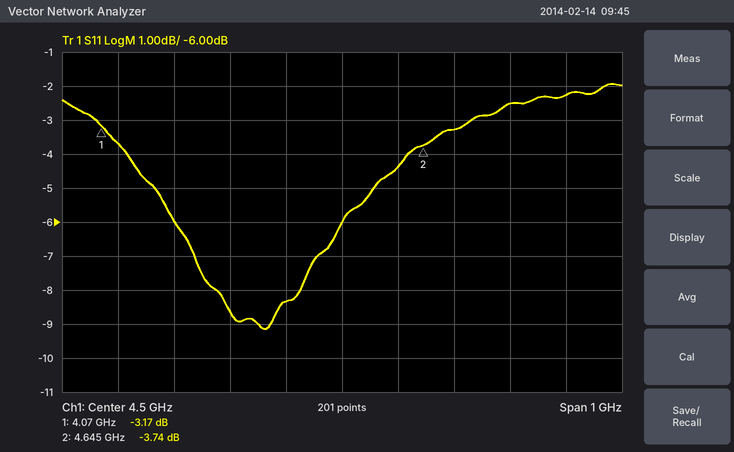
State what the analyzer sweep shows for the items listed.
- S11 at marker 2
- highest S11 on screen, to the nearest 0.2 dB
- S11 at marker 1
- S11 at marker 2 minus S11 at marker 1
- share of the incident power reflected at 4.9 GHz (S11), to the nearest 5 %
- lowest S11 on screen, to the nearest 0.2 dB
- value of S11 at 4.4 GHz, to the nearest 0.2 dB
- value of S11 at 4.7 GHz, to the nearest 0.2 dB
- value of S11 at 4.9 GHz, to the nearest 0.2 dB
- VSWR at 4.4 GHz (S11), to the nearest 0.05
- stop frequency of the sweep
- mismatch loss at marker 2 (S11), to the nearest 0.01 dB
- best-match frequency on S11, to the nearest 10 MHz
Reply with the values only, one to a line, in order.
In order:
-3.74 dB
-2.0 dB
-3.17 dB
-0.57 dB
60 %
-9.2 dB
-8.4 dB
-3.2 dB
-2.2 dB
2.25
5 GHz
2.39 dB
4.36 GHz
